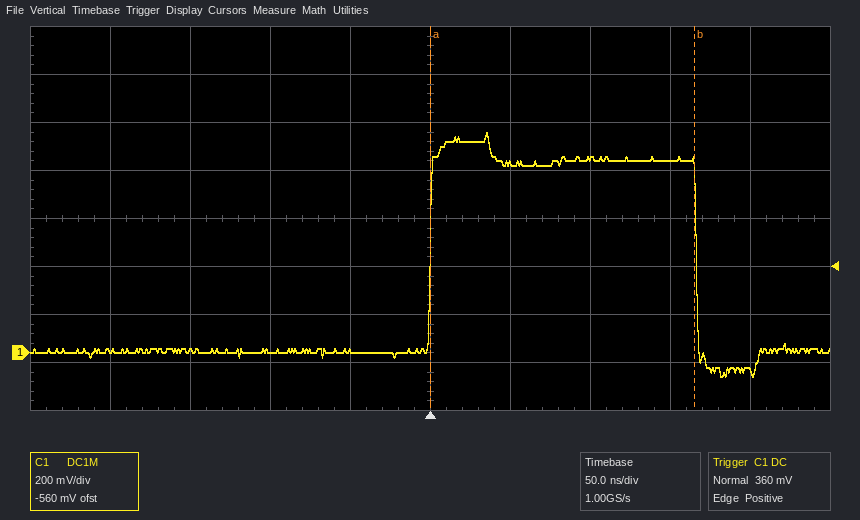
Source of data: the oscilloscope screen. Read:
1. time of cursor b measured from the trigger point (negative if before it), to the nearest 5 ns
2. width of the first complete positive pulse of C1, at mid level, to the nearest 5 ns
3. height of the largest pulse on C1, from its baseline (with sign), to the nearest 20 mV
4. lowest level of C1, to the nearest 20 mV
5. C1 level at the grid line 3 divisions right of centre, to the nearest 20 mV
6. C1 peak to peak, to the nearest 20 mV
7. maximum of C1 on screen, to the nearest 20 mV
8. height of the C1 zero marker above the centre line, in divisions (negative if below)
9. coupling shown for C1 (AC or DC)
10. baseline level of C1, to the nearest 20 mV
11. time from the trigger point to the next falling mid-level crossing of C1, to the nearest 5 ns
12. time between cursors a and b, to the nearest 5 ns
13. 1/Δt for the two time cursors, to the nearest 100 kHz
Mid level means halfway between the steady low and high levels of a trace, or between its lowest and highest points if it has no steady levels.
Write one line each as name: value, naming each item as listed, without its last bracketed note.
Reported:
time of cursor b measured from the trigger point (negative if before it), to the nearest 5 ns: +165 ns
width of the first complete positive pulse of C1, at mid level, to the nearest 5 ns: 165 ns
height of the largest pulse on C1, from its baseline (with sign), to the nearest 20 mV: +920 mV
lowest level of C1, to the nearest 20 mV: -100 mV
C1 level at the grid line 3 divisions right of centre, to the nearest 20 mV: 800 mV
C1 peak to peak, to the nearest 20 mV: 1.02 V
maximum of C1 on screen, to the nearest 20 mV: 920 mV
height of the C1 zero marker above the centre line, in divisions: -2.8 div
coupling shown for C1: DC
baseline level of C1, to the nearest 20 mV: 0 mV
time from the trigger point to the next falling mid-level crossing of C1, to the nearest 5 ns: 165 ns
time between cursors a and b, to the nearest 5 ns: 165 ns
1/Δt for the two time cursors, to the nearest 100 kHz: 6.1 MHz
